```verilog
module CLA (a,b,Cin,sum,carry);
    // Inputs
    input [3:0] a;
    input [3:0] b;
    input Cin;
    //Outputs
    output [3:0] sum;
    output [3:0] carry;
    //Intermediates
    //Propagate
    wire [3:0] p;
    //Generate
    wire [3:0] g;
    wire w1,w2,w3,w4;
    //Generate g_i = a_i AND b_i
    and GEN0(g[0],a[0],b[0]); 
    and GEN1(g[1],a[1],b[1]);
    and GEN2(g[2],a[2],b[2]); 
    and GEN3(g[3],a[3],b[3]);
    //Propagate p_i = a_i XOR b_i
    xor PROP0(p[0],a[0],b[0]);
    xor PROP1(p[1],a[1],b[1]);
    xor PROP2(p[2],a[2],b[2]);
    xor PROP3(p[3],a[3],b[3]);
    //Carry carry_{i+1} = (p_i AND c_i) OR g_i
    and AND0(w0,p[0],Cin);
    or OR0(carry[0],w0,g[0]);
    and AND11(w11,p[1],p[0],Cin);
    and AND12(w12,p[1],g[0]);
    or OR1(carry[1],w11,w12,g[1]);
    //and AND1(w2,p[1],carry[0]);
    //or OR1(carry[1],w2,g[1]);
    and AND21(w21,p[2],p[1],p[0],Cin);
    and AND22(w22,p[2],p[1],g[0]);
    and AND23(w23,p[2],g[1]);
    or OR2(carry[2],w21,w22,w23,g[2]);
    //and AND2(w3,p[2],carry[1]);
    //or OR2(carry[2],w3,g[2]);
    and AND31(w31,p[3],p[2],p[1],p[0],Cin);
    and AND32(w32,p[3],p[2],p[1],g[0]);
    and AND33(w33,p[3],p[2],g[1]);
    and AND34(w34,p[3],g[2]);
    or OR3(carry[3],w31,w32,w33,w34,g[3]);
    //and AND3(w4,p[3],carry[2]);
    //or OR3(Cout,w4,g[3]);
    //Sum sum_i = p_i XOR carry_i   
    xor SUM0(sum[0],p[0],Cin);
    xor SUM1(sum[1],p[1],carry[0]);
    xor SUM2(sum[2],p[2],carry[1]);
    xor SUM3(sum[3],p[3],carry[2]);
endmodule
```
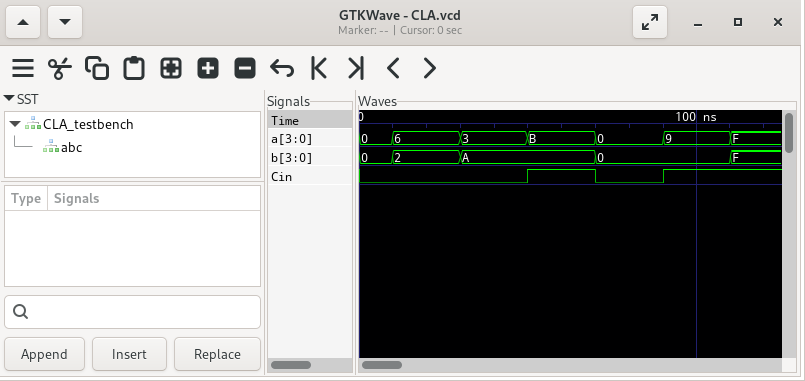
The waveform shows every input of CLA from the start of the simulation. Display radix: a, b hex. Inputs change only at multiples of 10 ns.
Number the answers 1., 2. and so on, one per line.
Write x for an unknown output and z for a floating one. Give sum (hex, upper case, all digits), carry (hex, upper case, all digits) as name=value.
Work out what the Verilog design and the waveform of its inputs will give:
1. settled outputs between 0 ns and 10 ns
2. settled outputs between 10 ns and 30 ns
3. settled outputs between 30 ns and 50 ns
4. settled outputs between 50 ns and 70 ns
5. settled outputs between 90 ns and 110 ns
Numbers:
1. sum=0, carry=0
2. sum=8, carry=6
3. sum=D, carry=2
4. sum=6, carry=B
5. sum=A, carry=1
